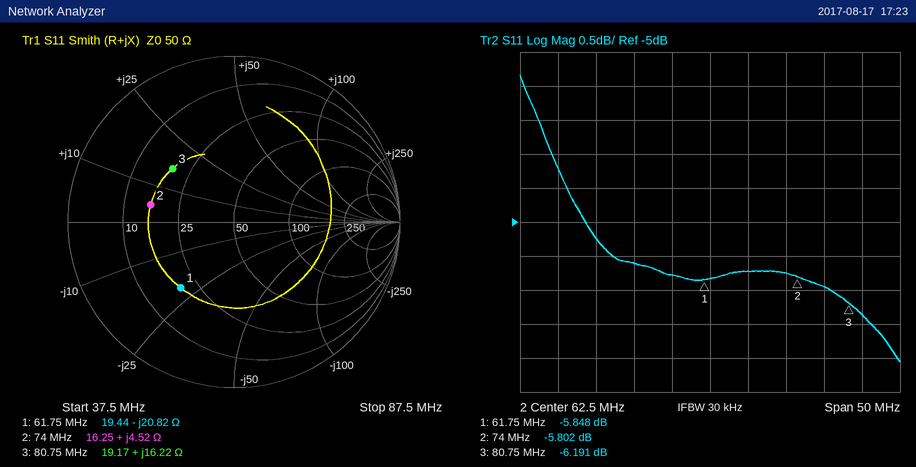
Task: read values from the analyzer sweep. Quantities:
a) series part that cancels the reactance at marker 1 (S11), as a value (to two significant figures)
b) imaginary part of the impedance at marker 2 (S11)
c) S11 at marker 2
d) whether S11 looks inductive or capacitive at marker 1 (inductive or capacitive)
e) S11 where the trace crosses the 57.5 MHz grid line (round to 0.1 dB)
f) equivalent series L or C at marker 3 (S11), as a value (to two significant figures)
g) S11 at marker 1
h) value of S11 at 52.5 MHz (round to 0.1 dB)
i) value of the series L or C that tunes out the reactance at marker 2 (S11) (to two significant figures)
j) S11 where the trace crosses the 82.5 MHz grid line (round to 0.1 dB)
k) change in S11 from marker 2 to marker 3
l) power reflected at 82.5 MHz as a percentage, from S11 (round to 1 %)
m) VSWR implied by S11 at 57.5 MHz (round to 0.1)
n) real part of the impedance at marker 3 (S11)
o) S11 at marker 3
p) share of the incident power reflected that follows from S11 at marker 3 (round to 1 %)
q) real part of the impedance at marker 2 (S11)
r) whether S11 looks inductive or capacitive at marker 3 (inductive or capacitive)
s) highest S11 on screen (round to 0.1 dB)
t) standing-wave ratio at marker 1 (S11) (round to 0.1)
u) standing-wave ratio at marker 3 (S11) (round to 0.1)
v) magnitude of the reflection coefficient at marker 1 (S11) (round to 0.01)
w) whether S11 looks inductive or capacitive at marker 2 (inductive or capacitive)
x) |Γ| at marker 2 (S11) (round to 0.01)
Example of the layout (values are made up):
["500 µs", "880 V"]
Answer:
["54 nH", "+4.52 Ω", "-5.802 dB", "capacitive", "-5.8 dB", "32 nH", "-5.848 dB", "-5.6 dB", "480 pF", "-6.4 dB", "-0.389 dB", "23 %", "3.1", "19.17 Ω", "-6.191 dB", "24 %", "16.25 Ω", "inductive", "-2.8 dB", "3.1", "2.9", "0.51", "inductive", "0.51"]
